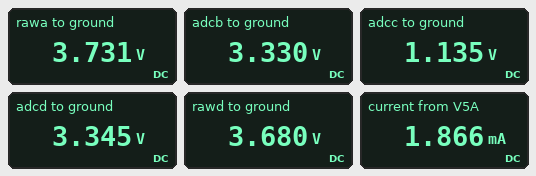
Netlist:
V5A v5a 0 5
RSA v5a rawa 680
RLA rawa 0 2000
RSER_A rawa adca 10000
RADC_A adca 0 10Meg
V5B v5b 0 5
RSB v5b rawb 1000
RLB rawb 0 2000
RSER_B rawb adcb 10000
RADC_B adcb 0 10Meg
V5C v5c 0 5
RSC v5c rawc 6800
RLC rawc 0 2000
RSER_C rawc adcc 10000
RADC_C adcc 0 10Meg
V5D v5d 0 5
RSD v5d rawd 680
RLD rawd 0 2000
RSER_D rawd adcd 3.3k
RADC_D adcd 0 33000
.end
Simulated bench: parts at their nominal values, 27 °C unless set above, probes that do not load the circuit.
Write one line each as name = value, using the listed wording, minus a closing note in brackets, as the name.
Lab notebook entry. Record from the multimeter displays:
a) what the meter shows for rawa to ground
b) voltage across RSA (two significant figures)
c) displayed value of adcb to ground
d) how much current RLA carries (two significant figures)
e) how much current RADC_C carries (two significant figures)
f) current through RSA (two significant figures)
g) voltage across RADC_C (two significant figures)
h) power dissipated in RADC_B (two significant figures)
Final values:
what the meter shows for rawa to ground = 3.731 V
voltage across RSA = 1.3 V
displayed value of adcb to ground = 3.330 V
how much current RLA carries = 1.9 mA
how much current RADC_C carries = 110 nA
current through RSA = 1.9 mA
voltage across RADC_C = 1.1 V
power dissipated in RADC_B = 1.1 µW
